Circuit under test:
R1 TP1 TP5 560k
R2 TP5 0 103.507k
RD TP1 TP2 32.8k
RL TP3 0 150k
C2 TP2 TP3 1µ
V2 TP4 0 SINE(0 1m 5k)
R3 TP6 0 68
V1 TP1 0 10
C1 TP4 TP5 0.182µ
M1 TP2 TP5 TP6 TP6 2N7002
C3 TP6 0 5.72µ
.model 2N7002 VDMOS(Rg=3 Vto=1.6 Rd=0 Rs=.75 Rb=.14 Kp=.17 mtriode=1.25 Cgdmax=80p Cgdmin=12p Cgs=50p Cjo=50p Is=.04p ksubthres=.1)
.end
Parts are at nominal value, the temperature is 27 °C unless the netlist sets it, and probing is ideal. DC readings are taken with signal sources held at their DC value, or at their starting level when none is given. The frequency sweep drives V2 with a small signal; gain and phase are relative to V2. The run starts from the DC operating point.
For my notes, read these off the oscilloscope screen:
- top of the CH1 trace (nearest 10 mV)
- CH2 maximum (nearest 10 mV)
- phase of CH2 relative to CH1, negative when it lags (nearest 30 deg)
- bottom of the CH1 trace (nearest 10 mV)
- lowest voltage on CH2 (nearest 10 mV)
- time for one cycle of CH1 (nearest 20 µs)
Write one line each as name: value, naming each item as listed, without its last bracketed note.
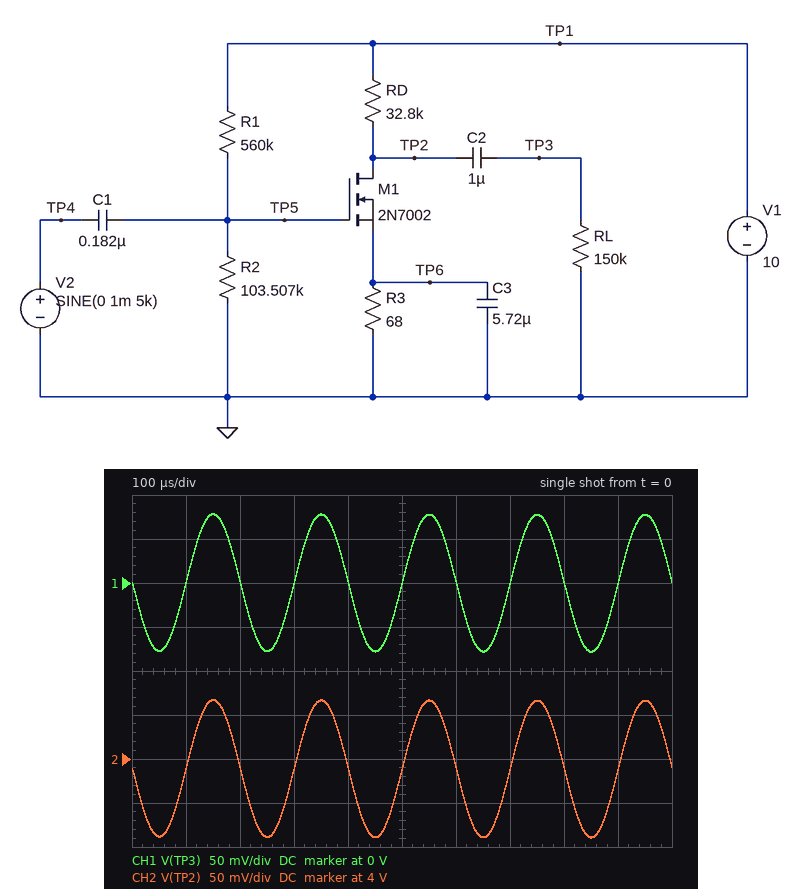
top of the CH1 trace: 80 mV
CH2 maximum: 4.07 V
phase of CH2 relative to CH1, negative when it lags: 0 deg
bottom of the CH1 trace: -80 mV
lowest voltage on CH2: 3.91 V
time for one cycle of CH1: 200 µs
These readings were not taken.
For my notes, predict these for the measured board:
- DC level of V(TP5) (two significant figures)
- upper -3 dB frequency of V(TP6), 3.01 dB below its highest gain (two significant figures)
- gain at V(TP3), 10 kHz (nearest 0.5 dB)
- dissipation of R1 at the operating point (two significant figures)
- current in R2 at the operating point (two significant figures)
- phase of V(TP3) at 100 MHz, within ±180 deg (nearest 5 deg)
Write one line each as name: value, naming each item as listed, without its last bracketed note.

DC level of V(TP5): 1.6 V
upper -3 dB frequency of V(TP6), 3.01 dB below its highest gain: 510 Hz
gain at V(TP3), 10 kHz: 38.0 dB
dissipation of R1 at the operating point: 130 µW
current in R2 at the operating point: 15 µA
phase of V(TP3) at 100 MHz, within ±180 deg: 5 deg
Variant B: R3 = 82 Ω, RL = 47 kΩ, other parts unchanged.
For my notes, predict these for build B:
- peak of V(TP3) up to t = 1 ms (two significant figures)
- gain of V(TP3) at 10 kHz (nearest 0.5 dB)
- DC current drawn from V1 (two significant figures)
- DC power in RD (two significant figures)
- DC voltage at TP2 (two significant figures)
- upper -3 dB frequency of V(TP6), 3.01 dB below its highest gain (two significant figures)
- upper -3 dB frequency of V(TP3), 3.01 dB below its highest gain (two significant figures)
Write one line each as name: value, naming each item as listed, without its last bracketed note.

peak of V(TP3) up to t = 1 ms: 55 mV
gain of V(TP3) at 10 kHz: 34.5 dB
DC current drawn from V1: 190 µA
DC power in RD: 1.0 mW
DC voltage at TP2: 4.2 V
upper -3 dB frequency of V(TP6), 3.01 dB below its highest gain: 440 Hz
upper -3 dB frequency of V(TP3), 3.01 dB below its highest gain: 200 kHz
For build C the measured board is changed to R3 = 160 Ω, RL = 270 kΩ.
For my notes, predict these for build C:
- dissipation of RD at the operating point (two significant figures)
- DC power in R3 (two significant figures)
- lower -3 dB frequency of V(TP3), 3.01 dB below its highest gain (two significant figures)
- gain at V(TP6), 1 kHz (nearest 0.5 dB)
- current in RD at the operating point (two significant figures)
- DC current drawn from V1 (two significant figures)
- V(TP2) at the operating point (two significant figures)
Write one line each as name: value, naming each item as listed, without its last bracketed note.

dissipation of RD at the operating point: 750 µW
DC power in R3: 3.7 µW
lower -3 dB frequency of V(TP3), 3.01 dB below its highest gain: 40 Hz
gain at V(TP6), 1 kHz: -23.5 dB
current in RD at the operating point: 150 µA
DC current drawn from V1: 170 µA
V(TP2) at the operating point: 5.0 V
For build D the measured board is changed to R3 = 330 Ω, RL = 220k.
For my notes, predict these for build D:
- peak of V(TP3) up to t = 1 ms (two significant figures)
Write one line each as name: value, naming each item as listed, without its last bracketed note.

peak of V(TP3) up to t = 1 ms: 56 mV
